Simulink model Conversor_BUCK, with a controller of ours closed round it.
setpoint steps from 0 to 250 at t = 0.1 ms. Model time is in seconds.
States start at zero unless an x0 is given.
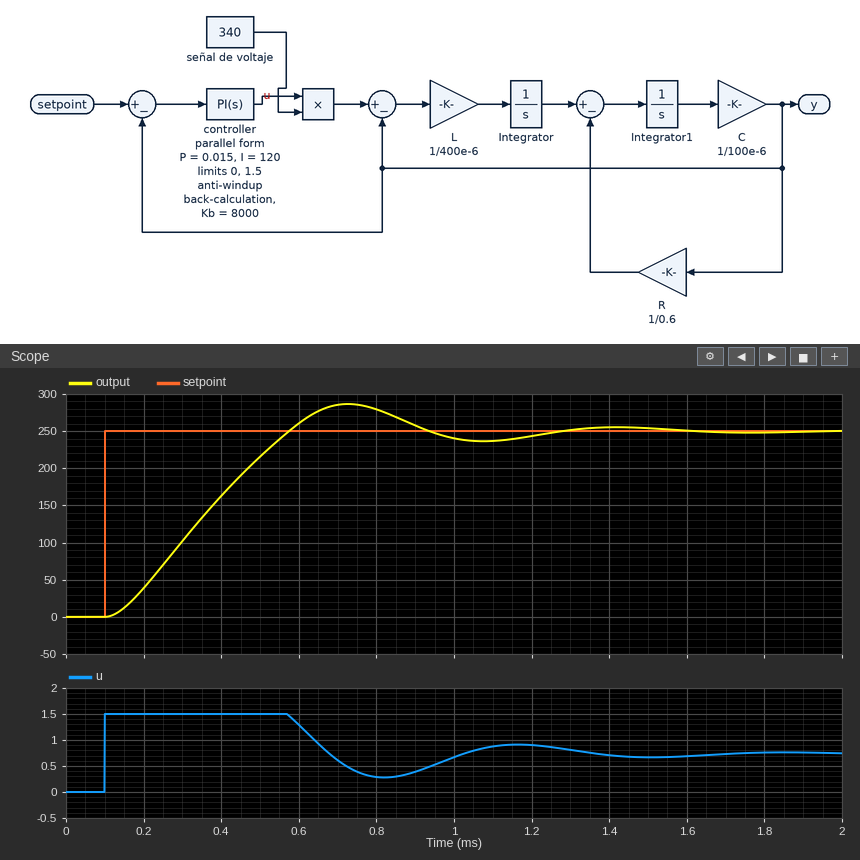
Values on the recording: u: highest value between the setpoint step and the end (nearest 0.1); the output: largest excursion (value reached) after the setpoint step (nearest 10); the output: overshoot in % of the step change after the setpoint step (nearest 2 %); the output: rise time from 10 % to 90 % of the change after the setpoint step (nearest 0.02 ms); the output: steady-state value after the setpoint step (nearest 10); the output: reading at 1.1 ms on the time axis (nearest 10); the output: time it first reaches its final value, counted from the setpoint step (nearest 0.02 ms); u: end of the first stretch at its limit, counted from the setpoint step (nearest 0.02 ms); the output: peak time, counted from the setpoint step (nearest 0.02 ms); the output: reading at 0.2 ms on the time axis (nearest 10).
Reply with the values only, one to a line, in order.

1.5
290
14 %
0.34 ms
250
240
0.48 ms
0.48 ms
0.62 ms
40
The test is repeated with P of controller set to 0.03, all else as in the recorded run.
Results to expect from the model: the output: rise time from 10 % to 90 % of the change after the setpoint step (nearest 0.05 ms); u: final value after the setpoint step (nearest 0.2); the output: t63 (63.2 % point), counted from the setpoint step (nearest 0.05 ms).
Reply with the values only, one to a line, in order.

0.35 ms
0.8
0.30 ms
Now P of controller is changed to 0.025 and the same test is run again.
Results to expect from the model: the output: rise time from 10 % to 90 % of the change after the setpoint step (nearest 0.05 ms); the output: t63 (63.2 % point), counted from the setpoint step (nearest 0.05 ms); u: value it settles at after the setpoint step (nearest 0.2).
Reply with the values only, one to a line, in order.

0.35 ms
0.30 ms
0.8
